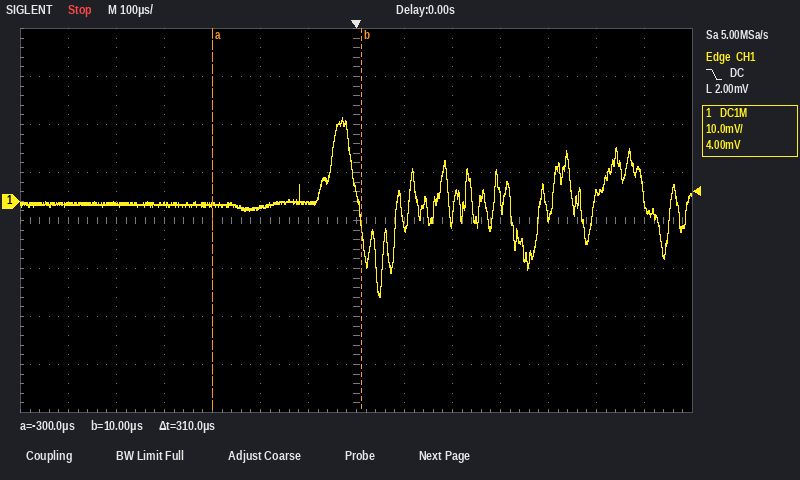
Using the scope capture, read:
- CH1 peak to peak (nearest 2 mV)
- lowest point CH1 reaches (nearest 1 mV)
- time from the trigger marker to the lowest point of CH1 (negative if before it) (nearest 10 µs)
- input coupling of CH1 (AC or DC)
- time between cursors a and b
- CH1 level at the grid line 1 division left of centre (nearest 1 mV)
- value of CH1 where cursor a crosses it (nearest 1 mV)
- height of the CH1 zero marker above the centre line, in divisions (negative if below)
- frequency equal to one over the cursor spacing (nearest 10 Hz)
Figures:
38 mV
-20 mV
+50 µs
DC
310 µs
0 mV
-1 mV
+0.4 div
3.23 kHz
